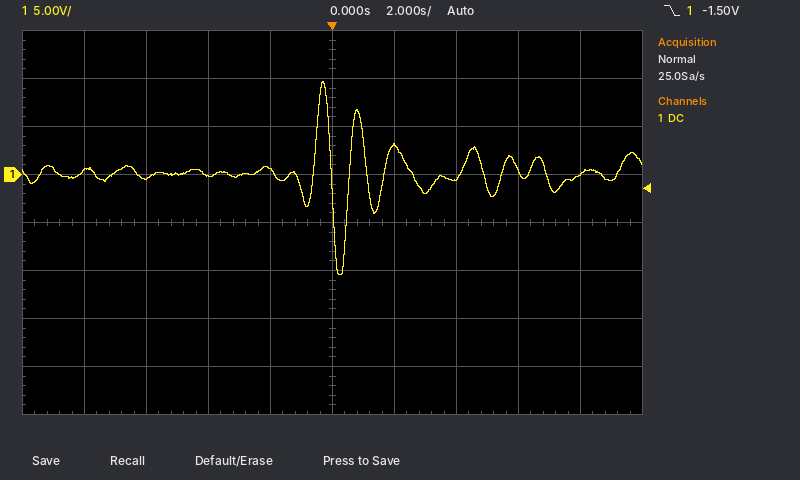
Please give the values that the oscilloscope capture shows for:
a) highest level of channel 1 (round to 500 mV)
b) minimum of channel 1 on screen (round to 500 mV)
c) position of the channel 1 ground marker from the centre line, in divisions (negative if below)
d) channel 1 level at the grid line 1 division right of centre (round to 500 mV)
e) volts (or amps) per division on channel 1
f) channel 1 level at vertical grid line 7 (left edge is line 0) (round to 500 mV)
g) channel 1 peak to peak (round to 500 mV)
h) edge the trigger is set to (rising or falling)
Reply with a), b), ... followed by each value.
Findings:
a) 9.5 V
b) -10.5 V
c) +1.0 div
d) 3.0 V
e) 5 V
f) -500 mV
g) 20.0 V
h) falling
